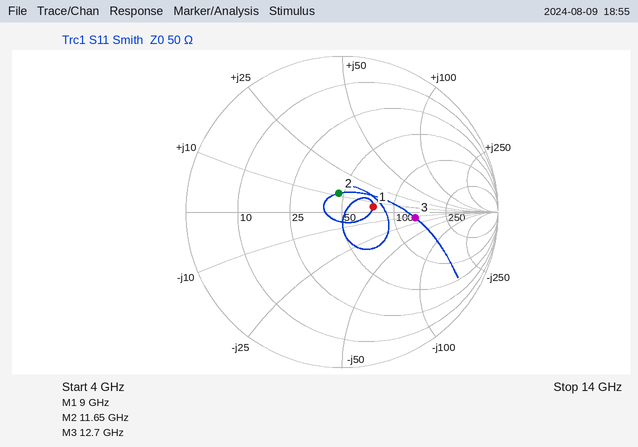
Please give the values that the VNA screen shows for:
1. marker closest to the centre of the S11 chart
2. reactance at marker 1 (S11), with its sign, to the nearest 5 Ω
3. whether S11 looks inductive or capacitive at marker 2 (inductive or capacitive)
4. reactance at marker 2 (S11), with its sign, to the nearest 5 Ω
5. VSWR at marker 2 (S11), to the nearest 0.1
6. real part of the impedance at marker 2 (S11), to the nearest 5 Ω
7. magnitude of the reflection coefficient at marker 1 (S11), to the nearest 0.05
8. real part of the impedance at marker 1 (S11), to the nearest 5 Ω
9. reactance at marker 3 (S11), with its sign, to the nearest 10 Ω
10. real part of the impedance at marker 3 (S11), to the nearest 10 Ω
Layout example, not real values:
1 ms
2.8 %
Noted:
marker 2
+5 Ω
inductive
+10 Ω
1.3
45 Ω
0.20
75 Ω
-10 Ω
140 Ω
